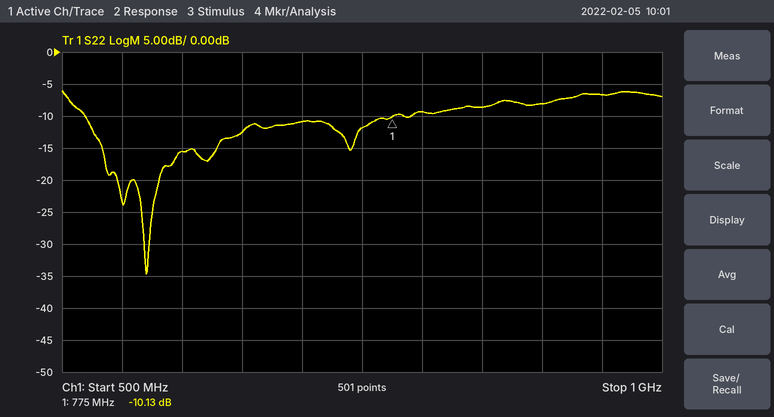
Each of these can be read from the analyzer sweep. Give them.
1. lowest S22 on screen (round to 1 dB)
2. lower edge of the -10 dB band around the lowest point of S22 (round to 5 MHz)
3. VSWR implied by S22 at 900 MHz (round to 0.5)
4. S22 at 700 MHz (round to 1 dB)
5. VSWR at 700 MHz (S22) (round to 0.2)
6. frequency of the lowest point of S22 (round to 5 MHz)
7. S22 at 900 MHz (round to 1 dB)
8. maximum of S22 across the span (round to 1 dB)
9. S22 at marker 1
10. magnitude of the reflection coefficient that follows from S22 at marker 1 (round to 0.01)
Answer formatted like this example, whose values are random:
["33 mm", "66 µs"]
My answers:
["-35 dB", "520 MHz", "2.5", "-11 dB", "1.8", "570 MHz", "-8 dB", "-6 dB", "-10.13 dB", "0.31"]
